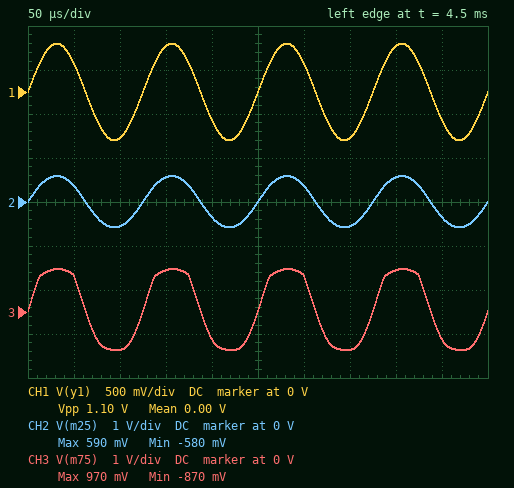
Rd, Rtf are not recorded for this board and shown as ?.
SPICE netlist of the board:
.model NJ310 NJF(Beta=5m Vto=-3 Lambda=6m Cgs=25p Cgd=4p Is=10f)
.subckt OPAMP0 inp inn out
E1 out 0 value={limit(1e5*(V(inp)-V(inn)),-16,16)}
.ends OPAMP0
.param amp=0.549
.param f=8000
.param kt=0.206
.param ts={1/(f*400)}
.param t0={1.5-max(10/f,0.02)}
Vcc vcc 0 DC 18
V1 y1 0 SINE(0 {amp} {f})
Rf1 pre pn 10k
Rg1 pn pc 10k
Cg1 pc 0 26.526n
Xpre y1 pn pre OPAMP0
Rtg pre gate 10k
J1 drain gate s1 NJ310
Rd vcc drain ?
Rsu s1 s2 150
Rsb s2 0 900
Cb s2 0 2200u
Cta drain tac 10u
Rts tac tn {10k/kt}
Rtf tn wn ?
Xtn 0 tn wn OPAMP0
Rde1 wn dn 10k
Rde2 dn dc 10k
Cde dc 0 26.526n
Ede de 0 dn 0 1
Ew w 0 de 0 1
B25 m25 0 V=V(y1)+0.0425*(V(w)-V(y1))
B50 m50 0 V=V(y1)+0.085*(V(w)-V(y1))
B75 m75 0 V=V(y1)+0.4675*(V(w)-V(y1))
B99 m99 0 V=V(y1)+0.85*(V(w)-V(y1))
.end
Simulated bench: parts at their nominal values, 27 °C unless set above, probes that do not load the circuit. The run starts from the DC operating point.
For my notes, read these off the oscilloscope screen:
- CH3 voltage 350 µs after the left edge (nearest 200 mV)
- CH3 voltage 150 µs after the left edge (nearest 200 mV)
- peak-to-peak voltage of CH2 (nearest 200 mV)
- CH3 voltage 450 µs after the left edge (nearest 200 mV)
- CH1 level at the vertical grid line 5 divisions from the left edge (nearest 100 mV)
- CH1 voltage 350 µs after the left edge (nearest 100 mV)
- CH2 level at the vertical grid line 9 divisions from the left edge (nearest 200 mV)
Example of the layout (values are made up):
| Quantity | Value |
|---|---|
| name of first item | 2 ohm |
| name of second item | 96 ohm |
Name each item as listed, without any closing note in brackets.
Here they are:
| Quantity | Value |
|---|---|
| CH3 voltage 350 µs after the left edge | -800 mV |
| CH3 voltage 150 µs after the left edge | 1.0 V |
| peak-to-peak voltage of CH2 | 1.2 V |
| CH3 voltage 450 µs after the left edge | -600 mV |
| CH1 level at the vertical grid line 5 divisions from the left edge | 0 V |
| CH1 voltage 350 µs after the left edge | -500 mV |
| CH2 level at the vertical grid line 9 divisions from the left edge | -400 mV |
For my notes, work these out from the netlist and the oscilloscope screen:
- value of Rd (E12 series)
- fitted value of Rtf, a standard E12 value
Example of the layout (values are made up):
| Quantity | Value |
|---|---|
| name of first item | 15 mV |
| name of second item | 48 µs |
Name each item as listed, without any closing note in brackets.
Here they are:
| Quantity | Value |
|---|---|
| value of Rd | 3.3 kΩ |
| fitted value of Rtf, a standard E12 value | 18 kΩ |
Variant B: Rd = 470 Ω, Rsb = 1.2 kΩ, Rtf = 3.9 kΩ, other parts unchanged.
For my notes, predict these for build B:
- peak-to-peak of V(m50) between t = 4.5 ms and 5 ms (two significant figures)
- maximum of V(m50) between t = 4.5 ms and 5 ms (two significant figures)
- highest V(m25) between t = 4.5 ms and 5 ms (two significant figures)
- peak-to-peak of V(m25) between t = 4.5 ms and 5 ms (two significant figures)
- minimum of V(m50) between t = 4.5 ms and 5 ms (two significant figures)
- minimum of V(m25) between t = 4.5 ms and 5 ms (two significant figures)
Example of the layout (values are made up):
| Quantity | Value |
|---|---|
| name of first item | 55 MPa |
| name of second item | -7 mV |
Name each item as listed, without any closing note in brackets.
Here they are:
| Quantity | Value |
|---|---|
| peak-to-peak of V(m50) between t = 4.5 ms and 5 ms | 1.0 V |
| maximum of V(m50) between t = 4.5 ms and 5 ms | 510 mV |
| highest V(m25) between t = 4.5 ms and 5 ms | 530 mV |
| peak-to-peak of V(m25) between t = 4.5 ms and 5 ms | 1.1 V |
| minimum of V(m50) between t = 4.5 ms and 5 ms | -500 mV |
| minimum of V(m25) between t = 4.5 ms and 5 ms | -530 mV |
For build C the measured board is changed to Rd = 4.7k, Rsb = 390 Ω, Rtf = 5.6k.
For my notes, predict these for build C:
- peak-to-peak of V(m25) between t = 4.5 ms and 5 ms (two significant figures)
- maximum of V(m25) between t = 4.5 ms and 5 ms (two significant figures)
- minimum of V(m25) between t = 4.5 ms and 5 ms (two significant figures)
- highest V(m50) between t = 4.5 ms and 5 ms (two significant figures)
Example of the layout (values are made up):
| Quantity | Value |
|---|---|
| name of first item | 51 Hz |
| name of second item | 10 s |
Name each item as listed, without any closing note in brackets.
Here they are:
| Quantity | Value |
|---|---|
| peak-to-peak of V(m25) between t = 4.5 ms and 5 ms | 1.1 V |
| maximum of V(m25) between t = 4.5 ms and 5 ms | 520 mV |
| minimum of V(m25) between t = 4.5 ms and 5 ms | -560 mV |
| highest V(m50) between t = 4.5 ms and 5 ms | 490 mV |
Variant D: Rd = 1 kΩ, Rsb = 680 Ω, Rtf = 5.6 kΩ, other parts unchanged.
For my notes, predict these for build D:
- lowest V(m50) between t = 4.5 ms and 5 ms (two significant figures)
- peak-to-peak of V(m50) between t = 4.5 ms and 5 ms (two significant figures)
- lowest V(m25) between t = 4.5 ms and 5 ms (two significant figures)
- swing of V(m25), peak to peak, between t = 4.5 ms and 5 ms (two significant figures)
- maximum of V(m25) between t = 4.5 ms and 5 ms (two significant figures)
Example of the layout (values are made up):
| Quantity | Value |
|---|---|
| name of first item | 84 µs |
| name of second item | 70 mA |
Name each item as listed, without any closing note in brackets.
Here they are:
| Quantity | Value |
|---|---|
| lowest V(m50) between t = 4.5 ms and 5 ms | -510 mV |
| peak-to-peak of V(m50) between t = 4.5 ms and 5 ms | 1.0 V |
| lowest V(m25) between t = 4.5 ms and 5 ms | -530 mV |
| swing of V(m25), peak to peak, between t = 4.5 ms and 5 ms | 1.1 V |
| maximum of V(m25) between t = 4.5 ms and 5 ms | 540 mV |
